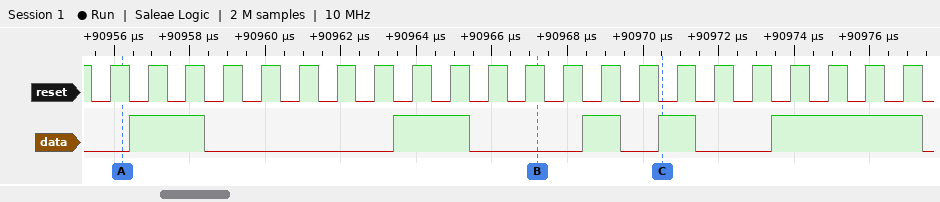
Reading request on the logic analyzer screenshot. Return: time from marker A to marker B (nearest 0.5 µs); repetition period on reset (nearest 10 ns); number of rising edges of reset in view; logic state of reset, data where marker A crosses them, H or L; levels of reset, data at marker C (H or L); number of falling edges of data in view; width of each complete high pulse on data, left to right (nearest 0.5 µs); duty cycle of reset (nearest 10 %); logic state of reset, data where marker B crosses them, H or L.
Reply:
11 µs
1000 ns
22
reset=H, data=L
reset=L, data=H
5
2 µs, 2 µs, 1 µs, 1 µs, 4 µs
50 %
reset=H, data=L
